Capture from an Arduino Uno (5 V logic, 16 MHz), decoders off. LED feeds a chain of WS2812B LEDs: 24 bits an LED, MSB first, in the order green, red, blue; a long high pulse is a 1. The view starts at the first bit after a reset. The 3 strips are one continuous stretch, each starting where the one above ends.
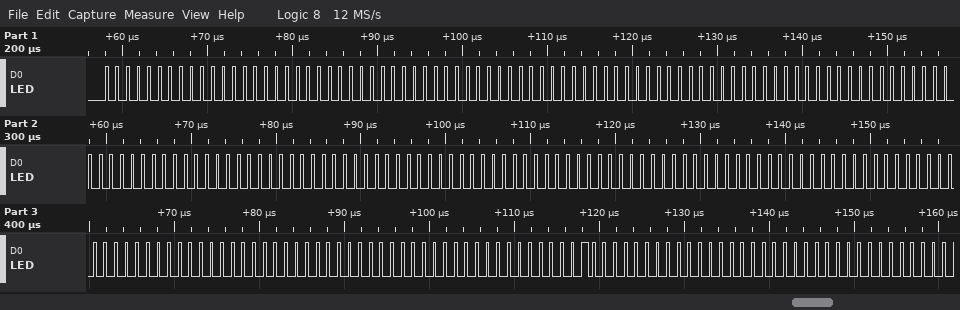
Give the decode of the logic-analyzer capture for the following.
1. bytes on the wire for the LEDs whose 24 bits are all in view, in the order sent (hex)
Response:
00 00 00 00 00 00 00 00 00 00 00 00 00 00 00 00 00 00 00 00 00 00 00 00 00 00 80 00 00 00
